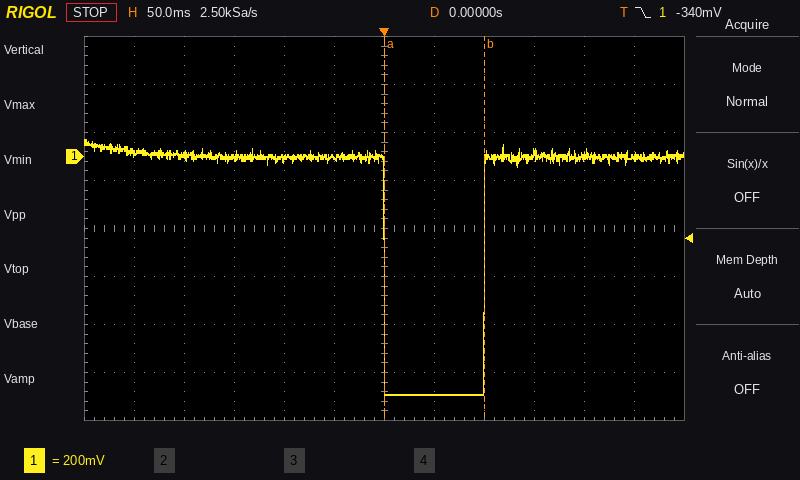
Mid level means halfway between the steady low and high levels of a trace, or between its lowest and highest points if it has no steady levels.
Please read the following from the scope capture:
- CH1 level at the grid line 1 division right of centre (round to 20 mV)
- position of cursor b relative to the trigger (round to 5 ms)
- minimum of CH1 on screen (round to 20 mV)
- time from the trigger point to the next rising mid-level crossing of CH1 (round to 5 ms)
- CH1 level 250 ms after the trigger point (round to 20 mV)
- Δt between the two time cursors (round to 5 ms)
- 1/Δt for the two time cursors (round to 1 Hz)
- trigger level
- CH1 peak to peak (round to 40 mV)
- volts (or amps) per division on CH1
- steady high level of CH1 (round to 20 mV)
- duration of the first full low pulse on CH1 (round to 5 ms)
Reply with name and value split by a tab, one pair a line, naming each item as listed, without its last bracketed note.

CH1 level at the grid line 1 division right of centre	-1.00 V
position of cursor b relative to the trigger	+100 ms
minimum of CH1 on screen	-1.00 V
time from the trigger point to the next rising mid-level crossing of CH1	100 ms
CH1 level 250 ms after the trigger point	0 mV
Δt between the two time cursors	100 ms
1/Δt for the two time cursors	10 Hz
trigger level	-340 mV
CH1 peak to peak	1.08 V
volts (or amps) per division on CH1	200 mV
steady high level of CH1	0 mV
duration of the first full low pulse on CH1	100 ms
